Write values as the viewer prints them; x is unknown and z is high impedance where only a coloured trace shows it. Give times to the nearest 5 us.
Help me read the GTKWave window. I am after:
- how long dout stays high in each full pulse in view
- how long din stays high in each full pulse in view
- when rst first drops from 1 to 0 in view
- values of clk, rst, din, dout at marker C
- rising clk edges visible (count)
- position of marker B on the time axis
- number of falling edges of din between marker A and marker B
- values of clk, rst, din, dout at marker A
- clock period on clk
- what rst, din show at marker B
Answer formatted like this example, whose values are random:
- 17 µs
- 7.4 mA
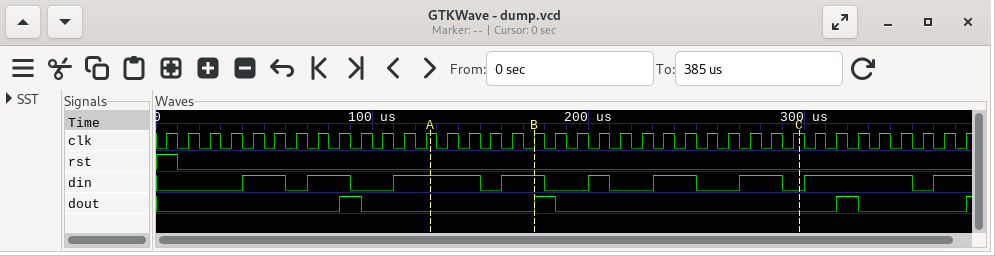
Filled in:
- 10 us, 10 us, 10 us
- 20 us, 20 us, 40 us, 20 us, 10 us, 20 us, 20 us, 50 us
- 10 us
- clk=1, rst=0, din=0, dout=0
- 38
- 175 us
- 1
- clk=1, rst=0, din=1, dout=0
- 10 us
- rst=0, din=1
